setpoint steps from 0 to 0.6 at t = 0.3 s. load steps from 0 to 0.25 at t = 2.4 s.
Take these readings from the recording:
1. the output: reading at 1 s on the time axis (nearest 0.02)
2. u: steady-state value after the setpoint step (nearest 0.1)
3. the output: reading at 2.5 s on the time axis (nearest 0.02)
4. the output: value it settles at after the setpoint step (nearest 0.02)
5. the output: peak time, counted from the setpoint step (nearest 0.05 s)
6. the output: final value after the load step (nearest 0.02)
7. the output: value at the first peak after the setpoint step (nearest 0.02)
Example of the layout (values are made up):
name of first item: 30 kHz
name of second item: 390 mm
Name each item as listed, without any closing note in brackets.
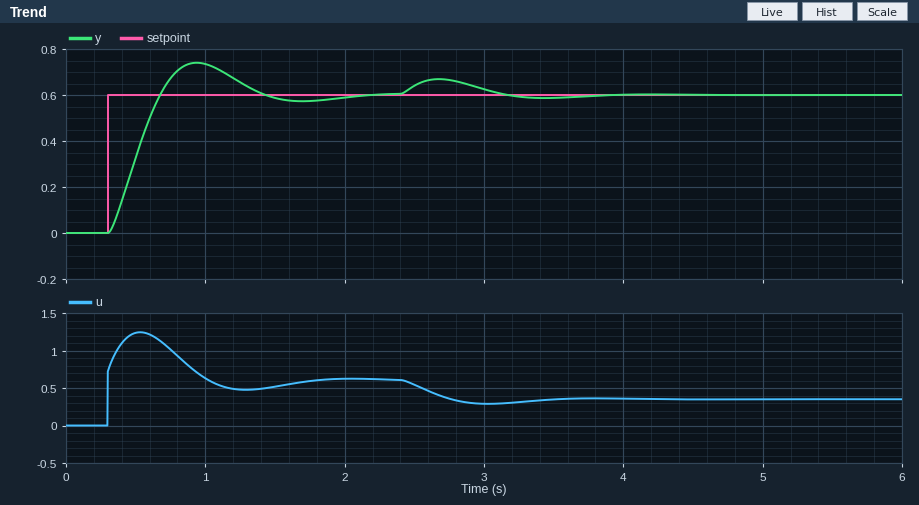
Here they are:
the output: reading at 1 s on the time axis: 0.74
u: steady-state value after the setpoint step: 0.6
the output: reading at 2.5 s on the time axis: 0.64
the output: value it settles at after the setpoint step: 0.60
the output: peak time, counted from the setpoint step: 0.65 s
the output: final value after the load step: 0.60
the output: value at the first peak after the setpoint step: 0.74
